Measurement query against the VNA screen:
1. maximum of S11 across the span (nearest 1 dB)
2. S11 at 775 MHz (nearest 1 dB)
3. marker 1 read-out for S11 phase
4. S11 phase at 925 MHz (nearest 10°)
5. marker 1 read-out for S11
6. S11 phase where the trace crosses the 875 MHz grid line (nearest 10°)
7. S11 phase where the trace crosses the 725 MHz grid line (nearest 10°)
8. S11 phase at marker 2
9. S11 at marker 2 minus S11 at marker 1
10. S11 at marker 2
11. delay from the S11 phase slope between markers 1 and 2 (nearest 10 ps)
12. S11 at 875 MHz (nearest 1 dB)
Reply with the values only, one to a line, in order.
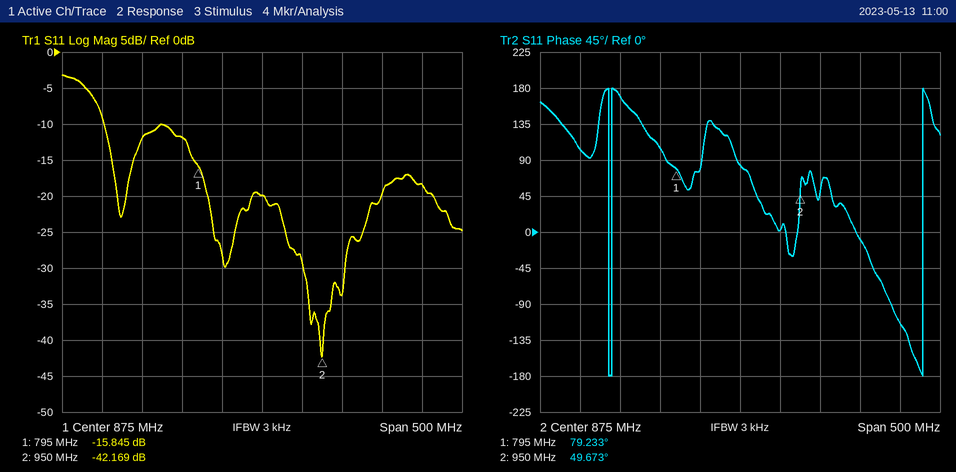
-3 dB
-12 dB
79.233°
0°
-15.845 dB
80°
170°
49.673°
-26.324 dB
-42.169 dB
530 ps
-20 dB
